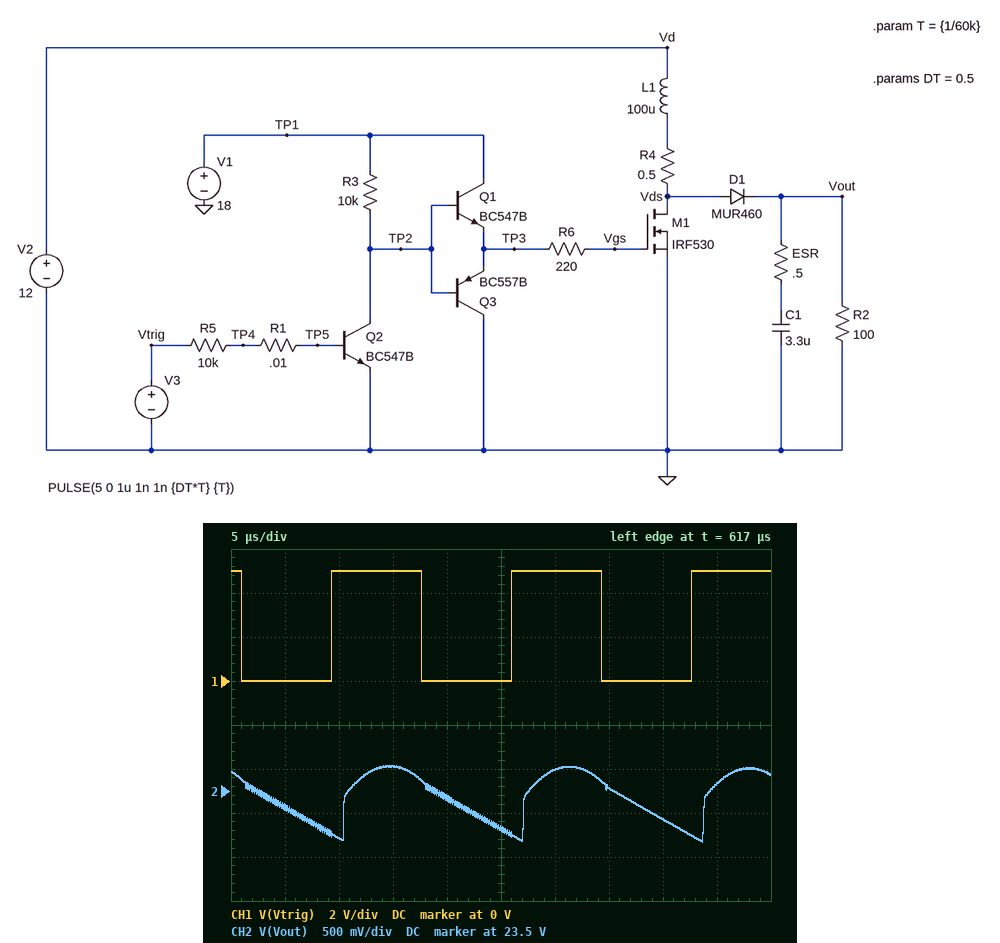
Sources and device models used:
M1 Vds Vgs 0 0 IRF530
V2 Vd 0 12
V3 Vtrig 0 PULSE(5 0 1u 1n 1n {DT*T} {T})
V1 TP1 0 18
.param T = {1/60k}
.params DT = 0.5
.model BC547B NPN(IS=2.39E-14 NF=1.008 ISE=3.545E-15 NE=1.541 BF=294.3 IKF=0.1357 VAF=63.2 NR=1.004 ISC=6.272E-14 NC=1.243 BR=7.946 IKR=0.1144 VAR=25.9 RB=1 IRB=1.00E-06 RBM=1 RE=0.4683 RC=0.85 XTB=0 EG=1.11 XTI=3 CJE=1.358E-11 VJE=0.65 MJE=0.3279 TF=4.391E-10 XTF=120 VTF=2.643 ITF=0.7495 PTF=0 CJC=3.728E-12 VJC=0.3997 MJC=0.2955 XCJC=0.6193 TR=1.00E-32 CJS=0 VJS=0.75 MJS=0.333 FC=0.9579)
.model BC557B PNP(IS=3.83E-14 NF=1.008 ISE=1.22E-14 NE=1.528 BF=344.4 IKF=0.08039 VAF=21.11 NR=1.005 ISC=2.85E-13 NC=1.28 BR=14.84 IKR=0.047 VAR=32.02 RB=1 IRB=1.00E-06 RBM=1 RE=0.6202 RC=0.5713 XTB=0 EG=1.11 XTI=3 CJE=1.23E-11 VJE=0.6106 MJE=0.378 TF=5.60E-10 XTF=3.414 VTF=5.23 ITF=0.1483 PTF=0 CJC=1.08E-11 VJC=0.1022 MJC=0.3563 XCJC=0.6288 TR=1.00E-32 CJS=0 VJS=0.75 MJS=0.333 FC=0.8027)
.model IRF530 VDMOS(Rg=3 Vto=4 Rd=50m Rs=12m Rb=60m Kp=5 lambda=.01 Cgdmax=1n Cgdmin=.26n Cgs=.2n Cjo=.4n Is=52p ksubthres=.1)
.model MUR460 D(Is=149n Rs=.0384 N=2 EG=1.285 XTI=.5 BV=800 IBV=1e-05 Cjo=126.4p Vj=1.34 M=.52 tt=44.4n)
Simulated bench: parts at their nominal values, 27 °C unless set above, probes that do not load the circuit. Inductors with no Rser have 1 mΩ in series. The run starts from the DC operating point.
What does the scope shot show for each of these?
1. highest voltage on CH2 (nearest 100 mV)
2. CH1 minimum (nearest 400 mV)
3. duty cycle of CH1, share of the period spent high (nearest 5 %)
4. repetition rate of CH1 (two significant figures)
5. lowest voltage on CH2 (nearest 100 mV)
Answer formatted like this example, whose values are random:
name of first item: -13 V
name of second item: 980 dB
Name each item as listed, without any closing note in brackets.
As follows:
highest voltage on CH2: 23.8 V
CH1 minimum: 0 V
duty cycle of CH1, share of the period spent high: 50 %
repetition rate of CH1: 60 kHz
lowest voltage on CH2: 22.9 V
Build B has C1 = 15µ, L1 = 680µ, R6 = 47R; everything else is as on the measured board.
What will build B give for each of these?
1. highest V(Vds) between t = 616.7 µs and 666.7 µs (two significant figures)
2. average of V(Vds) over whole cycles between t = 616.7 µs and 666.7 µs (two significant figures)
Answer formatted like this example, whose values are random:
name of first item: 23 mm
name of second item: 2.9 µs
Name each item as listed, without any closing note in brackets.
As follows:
highest V(Vds) between t = 616.7 µs and 666.7 µs: 29 V
average of V(Vds) over whole cycles between t = 616.7 µs and 666.7 µs: 15 V
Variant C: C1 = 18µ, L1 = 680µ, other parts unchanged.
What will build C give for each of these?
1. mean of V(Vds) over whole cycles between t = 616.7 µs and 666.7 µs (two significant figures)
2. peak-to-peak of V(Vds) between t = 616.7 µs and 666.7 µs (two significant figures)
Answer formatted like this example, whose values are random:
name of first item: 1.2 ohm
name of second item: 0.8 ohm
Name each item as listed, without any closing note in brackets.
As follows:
mean of V(Vds) over whole cycles between t = 616.7 µs and 666.7 µs: 14 V
peak-to-peak of V(Vds) between t = 616.7 µs and 666.7 µs: 30 V
